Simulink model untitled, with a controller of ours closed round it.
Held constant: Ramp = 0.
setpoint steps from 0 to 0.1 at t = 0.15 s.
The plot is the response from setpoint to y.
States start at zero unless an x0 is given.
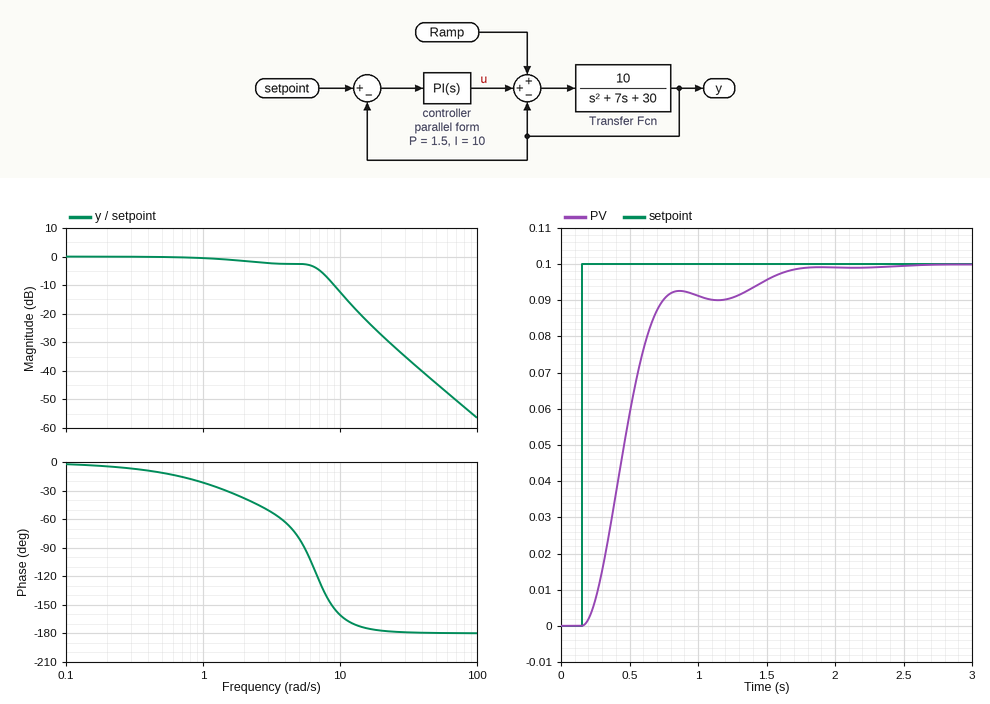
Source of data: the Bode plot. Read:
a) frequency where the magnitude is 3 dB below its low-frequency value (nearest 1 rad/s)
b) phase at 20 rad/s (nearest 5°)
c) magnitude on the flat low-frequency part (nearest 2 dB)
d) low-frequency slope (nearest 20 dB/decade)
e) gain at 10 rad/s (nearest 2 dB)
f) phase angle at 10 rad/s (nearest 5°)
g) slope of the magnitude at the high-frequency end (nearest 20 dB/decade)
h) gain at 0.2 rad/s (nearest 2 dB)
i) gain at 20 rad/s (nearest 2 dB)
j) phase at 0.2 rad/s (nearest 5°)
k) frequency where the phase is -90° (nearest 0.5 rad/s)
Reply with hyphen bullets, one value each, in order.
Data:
- 6 rad/s
- -175°
- 0 dB
- 0 dB/decade
- -12 dB
- -160°
- -40 dB/decade
- 0 dB
- -28 dB
- -5°
- 5.5 rad/s
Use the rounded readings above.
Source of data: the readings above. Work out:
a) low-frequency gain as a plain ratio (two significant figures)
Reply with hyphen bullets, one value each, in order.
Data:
- 1.0
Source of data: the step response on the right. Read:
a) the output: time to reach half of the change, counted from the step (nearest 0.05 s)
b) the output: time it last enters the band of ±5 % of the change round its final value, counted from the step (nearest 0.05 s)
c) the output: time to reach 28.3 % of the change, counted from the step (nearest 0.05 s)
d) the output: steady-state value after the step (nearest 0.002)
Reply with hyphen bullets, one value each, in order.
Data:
- 0.30 s
- 1.30 s
- 0.20 s
- 0.100
